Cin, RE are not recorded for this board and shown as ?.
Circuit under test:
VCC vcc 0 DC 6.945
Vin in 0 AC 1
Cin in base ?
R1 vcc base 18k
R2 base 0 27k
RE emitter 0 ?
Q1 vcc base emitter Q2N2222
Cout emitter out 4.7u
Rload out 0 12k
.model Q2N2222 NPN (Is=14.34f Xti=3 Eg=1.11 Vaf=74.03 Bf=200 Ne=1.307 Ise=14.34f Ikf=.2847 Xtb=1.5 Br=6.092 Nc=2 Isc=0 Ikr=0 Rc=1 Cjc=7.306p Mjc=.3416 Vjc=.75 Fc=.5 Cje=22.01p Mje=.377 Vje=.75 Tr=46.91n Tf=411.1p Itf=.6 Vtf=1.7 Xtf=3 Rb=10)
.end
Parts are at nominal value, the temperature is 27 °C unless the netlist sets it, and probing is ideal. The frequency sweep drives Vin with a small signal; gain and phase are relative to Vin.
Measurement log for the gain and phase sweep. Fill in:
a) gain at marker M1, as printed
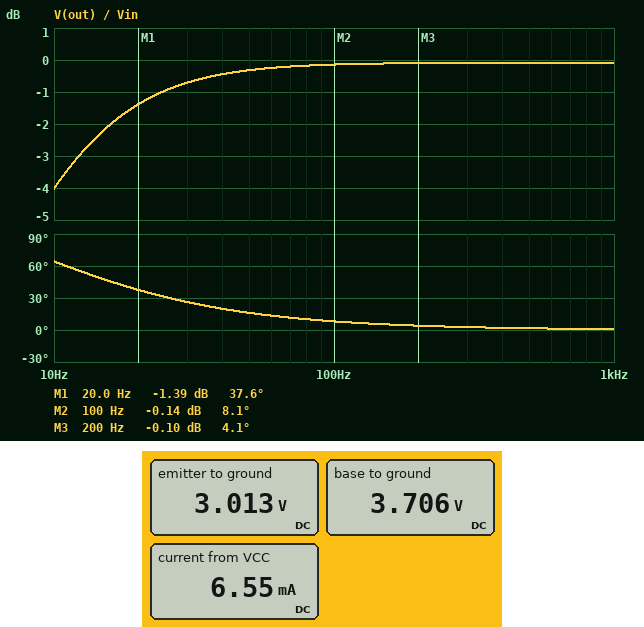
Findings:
-1.39 dB
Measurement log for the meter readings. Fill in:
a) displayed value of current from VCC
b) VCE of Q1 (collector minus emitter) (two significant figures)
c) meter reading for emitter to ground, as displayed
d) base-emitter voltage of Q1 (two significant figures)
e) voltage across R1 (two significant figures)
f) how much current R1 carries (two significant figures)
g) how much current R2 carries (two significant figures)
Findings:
6.55 mA
3.9 V
3.013 V
690 mV
3.2 V
180 µA
140 µA
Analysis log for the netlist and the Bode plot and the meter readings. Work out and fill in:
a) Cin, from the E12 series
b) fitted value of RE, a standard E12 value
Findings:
1.5 µF
470 Ω
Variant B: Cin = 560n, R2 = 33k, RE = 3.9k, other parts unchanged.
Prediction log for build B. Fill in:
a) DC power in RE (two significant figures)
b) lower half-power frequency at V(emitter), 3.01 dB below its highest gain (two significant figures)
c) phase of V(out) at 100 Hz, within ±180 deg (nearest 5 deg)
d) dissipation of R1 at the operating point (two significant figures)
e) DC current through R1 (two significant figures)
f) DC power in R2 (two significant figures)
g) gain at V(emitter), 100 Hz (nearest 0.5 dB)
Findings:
3.6 mW
25 Hz
15 deg
360 µW
140 µA
590 µW
-0.5 dB
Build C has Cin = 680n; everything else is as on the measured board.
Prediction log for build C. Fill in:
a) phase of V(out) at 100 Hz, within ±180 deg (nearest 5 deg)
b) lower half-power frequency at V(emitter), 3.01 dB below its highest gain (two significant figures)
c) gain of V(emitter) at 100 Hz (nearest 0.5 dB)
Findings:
15 deg
25 Hz
-0.5 dB
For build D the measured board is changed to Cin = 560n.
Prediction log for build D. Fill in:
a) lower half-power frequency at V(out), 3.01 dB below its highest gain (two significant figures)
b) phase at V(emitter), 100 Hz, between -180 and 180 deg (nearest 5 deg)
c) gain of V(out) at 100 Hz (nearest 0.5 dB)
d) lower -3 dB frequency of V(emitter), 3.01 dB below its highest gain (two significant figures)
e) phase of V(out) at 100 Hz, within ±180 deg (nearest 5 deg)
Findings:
31 Hz
15 deg
-0.5 dB
30 Hz
20 deg
